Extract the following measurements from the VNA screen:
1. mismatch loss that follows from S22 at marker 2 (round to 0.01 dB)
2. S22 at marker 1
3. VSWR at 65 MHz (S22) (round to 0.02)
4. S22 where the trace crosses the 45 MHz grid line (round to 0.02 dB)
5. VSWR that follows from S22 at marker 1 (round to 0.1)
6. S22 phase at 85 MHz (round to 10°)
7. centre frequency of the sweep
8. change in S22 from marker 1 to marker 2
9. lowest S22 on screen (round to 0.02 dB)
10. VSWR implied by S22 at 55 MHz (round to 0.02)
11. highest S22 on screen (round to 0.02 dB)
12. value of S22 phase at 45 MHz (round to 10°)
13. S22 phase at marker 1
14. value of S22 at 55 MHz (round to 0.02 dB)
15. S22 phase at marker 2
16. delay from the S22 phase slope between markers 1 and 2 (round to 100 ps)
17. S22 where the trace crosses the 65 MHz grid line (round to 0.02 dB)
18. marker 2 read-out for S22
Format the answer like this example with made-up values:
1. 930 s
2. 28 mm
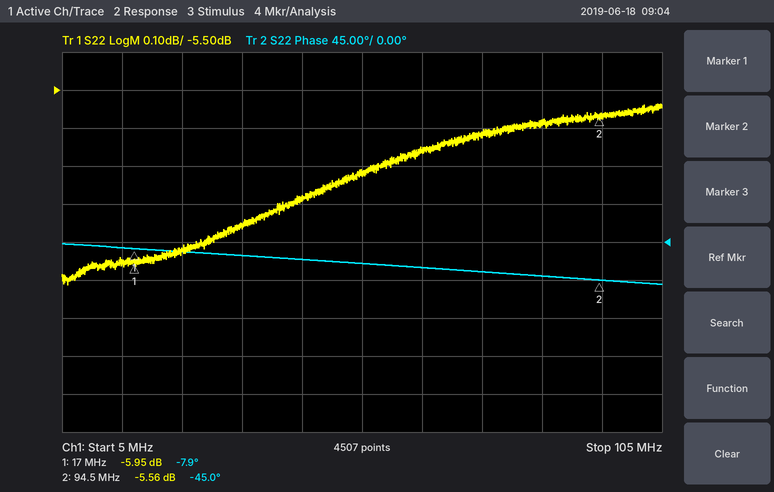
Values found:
1. 1.41 dB
2. -5.95 dB
3. 3.18
4. -5.78 dB
5. 3.0
6. -40°
7. 55 MHz
8. 0.39 dB
9. -6.02 dB
10. 3.14
11. -5.54 dB
12. -20°
13. -7.9°
14. -5.72 dB
15. -45.0°
16. 1.3 ns
17. -5.66 dB
18. -5.56 dB
